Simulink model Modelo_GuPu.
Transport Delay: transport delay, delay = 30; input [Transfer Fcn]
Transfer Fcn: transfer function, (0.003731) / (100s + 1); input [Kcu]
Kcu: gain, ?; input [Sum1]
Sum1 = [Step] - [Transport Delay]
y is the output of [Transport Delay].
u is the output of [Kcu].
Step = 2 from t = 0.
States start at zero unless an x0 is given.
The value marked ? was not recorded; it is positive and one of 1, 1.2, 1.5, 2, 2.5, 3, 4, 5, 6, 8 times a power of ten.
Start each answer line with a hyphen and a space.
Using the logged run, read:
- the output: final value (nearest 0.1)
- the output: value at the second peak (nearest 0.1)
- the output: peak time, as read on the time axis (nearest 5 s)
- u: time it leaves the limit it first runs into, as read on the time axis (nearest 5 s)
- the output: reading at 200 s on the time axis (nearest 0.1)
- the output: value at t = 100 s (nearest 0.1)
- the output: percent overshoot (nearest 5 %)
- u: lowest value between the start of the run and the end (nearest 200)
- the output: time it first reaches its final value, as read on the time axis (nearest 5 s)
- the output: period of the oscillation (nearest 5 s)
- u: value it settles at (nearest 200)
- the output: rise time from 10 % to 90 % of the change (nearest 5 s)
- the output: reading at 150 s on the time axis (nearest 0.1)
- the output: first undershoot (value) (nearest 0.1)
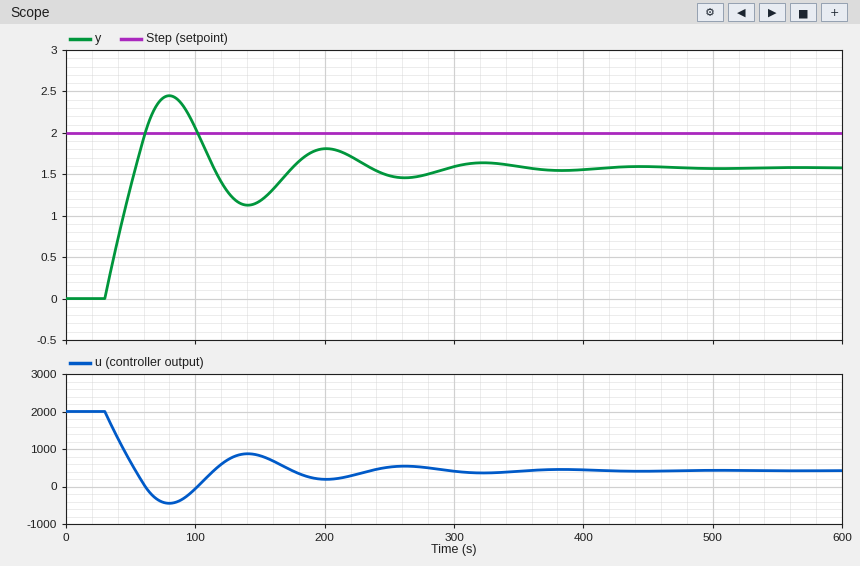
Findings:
- 1.6
- 1.8
- 80 s
- 30 s
- 1.8
- 2.1
- 55 %
- -400
- 55 s
- 120 s
- 400
- 20 s
- 1.2
- 1.1
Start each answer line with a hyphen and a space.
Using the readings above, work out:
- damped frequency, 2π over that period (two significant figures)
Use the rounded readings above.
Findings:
- 0.052 rad/s
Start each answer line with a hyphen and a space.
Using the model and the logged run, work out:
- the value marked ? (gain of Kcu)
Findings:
- 1000
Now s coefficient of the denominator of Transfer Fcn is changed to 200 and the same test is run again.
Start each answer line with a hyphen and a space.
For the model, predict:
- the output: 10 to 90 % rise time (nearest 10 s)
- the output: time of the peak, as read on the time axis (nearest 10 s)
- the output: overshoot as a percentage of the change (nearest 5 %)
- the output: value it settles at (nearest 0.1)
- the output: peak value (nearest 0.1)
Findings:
- 40 s
- 110 s
- 10 %
- 1.6
- 1.7
